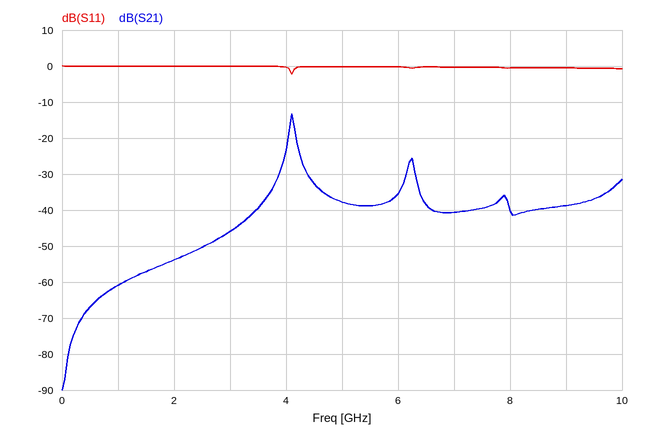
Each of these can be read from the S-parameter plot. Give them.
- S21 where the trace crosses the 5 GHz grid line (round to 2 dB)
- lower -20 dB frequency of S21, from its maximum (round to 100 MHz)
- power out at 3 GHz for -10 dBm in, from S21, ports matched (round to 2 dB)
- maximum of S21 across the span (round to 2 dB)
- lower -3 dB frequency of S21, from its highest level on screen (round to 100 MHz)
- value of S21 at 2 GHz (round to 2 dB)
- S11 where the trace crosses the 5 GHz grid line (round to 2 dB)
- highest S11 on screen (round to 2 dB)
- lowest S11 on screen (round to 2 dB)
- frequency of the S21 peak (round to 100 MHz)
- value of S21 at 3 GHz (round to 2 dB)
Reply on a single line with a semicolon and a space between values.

-38 dB; 3.8 GHz; -56 dBm; -14 dB; 4.1 GHz; -54 dB; 0 dB; 0 dB; -2 dB; 4.1 GHz; -46 dB
